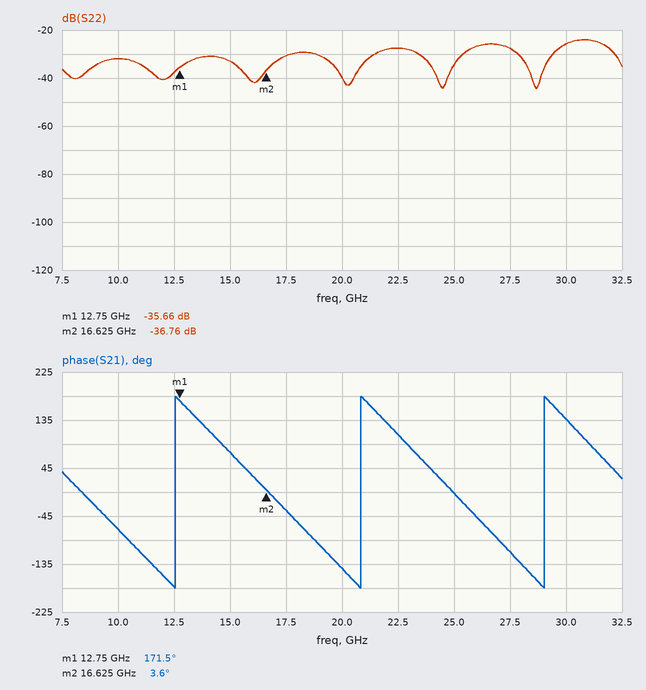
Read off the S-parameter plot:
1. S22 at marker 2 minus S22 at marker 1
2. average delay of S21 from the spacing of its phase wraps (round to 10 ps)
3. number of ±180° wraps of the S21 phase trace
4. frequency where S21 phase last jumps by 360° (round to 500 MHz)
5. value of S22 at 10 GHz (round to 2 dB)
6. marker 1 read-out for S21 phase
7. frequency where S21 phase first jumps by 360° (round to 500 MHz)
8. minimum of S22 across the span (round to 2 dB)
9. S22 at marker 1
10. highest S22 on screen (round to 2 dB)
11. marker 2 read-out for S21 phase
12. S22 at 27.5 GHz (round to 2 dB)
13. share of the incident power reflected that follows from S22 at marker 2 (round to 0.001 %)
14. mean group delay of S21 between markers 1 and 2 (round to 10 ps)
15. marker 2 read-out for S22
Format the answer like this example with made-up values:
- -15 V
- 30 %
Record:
- -1.10 dB
- 120 ps
- 3
- 29.0 GHz
- -32 dB
- 171.5°
- 12.5 GHz
- -44 dB
- -35.66 dB
- -24 dB
- 3.6°
- -28 dB
- 0.021 %
- 120 ps
- -36.76 dB
